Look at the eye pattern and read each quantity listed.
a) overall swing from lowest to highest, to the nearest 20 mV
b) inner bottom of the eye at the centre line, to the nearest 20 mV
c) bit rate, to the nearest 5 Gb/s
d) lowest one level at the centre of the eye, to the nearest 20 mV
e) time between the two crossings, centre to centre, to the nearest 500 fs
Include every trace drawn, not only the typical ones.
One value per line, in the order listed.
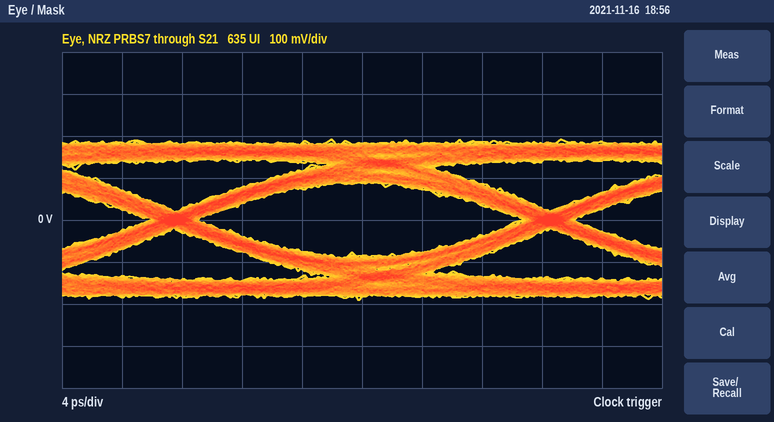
380 mV
-80 mV
40 Gb/s
80 mV
25.0 ps
